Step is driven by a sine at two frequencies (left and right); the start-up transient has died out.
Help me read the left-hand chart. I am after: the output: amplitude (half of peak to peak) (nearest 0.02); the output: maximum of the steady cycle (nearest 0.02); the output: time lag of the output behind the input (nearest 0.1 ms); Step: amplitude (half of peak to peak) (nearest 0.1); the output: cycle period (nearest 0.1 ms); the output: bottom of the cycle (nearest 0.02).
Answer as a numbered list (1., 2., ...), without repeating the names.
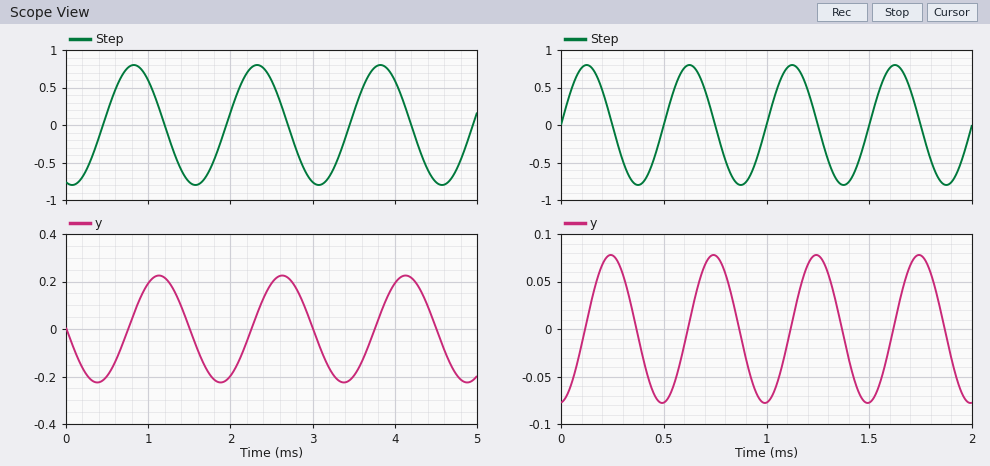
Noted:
1. 0.22
2. 0.22
3. 0.3 ms
4. 0.8
5. 1.5 ms
6. -0.22
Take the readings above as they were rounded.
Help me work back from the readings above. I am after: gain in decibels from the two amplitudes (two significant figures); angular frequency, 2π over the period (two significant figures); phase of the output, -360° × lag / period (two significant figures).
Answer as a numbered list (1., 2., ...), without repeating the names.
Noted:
1. -11 dB
2. 4.2 rad/ms
3. -72°
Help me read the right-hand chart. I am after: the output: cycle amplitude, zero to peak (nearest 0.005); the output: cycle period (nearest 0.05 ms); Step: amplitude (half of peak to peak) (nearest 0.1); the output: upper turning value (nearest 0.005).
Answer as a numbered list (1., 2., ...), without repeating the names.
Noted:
1. 0.080
2. 0.50 ms
3. 0.8
4. 0.080
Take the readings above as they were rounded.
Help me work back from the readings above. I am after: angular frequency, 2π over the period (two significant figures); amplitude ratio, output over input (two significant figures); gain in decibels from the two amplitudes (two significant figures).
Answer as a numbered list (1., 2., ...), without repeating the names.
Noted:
1. 13 rad/ms
2. 0.10
3. -20 dB
